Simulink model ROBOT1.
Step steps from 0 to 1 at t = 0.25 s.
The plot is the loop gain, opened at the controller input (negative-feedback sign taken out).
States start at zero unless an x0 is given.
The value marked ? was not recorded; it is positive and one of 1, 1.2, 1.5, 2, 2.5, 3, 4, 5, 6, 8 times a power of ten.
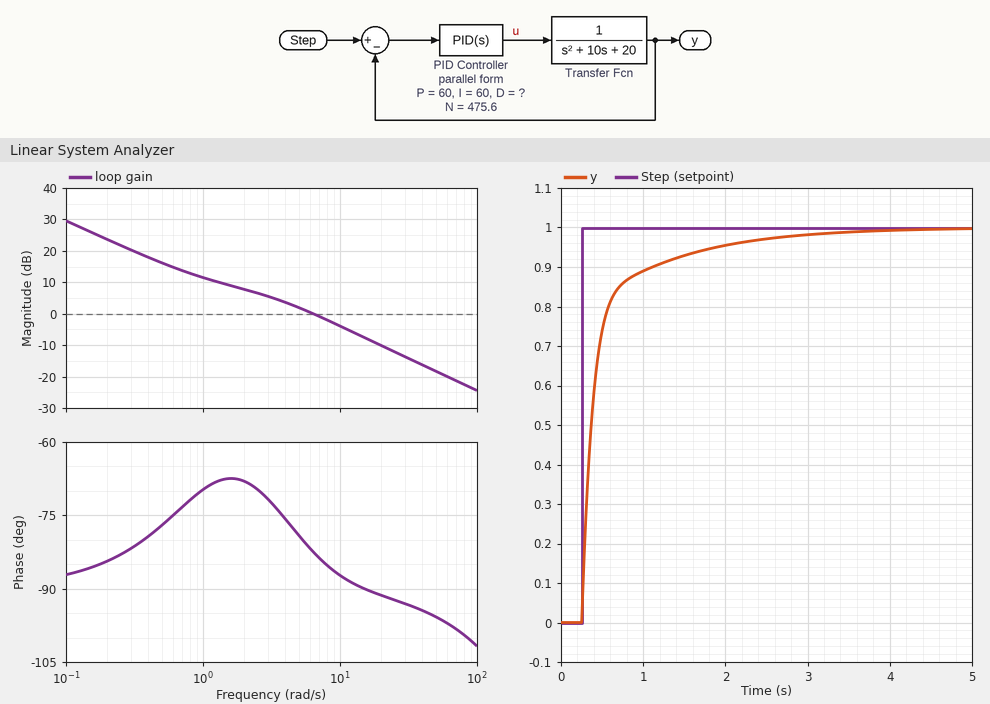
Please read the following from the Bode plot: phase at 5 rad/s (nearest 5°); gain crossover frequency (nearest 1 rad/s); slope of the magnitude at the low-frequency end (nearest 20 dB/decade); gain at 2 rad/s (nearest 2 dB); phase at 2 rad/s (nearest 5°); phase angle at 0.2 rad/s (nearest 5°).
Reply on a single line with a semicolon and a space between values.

-80°; 6 rad/s; -20 dB/decade; 8 dB; -70°; -85°
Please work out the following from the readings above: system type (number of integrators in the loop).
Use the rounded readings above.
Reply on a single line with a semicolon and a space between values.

1
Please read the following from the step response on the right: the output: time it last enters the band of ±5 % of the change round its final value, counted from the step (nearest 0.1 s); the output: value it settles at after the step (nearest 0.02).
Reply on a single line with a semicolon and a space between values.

1.6 s; 1.00
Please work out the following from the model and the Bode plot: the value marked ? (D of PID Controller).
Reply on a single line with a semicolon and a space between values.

6
